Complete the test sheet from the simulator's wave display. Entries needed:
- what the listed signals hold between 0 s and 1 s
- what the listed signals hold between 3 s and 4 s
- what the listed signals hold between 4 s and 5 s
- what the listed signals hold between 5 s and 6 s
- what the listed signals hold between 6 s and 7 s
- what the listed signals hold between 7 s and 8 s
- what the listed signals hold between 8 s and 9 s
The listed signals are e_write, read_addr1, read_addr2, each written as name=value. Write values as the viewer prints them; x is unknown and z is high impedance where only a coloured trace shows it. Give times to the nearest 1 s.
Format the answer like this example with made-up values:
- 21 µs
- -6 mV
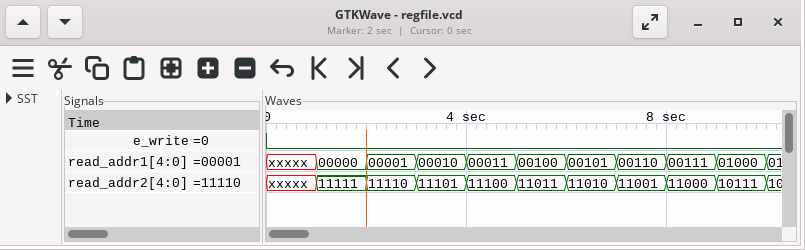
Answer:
- e_write=0, read_addr1=xxxxx, read_addr2=xxxxx
- e_write=0, read_addr1=00010, read_addr2=11101
- e_write=0, read_addr1=00011, read_addr2=11100
- e_write=0, read_addr1=00100, read_addr2=11011
- e_write=0, read_addr1=00101, read_addr2=11010
- e_write=0, read_addr1=00110, read_addr2=11001
- e_write=0, read_addr1=00111, read_addr2=11000
